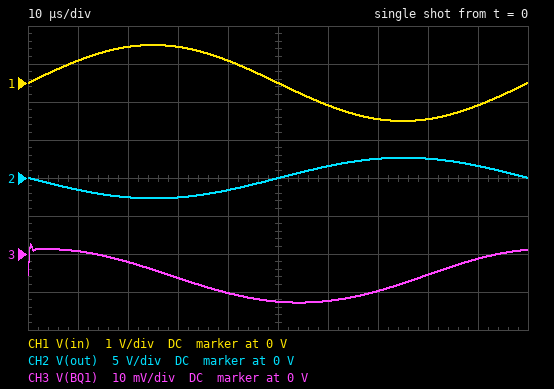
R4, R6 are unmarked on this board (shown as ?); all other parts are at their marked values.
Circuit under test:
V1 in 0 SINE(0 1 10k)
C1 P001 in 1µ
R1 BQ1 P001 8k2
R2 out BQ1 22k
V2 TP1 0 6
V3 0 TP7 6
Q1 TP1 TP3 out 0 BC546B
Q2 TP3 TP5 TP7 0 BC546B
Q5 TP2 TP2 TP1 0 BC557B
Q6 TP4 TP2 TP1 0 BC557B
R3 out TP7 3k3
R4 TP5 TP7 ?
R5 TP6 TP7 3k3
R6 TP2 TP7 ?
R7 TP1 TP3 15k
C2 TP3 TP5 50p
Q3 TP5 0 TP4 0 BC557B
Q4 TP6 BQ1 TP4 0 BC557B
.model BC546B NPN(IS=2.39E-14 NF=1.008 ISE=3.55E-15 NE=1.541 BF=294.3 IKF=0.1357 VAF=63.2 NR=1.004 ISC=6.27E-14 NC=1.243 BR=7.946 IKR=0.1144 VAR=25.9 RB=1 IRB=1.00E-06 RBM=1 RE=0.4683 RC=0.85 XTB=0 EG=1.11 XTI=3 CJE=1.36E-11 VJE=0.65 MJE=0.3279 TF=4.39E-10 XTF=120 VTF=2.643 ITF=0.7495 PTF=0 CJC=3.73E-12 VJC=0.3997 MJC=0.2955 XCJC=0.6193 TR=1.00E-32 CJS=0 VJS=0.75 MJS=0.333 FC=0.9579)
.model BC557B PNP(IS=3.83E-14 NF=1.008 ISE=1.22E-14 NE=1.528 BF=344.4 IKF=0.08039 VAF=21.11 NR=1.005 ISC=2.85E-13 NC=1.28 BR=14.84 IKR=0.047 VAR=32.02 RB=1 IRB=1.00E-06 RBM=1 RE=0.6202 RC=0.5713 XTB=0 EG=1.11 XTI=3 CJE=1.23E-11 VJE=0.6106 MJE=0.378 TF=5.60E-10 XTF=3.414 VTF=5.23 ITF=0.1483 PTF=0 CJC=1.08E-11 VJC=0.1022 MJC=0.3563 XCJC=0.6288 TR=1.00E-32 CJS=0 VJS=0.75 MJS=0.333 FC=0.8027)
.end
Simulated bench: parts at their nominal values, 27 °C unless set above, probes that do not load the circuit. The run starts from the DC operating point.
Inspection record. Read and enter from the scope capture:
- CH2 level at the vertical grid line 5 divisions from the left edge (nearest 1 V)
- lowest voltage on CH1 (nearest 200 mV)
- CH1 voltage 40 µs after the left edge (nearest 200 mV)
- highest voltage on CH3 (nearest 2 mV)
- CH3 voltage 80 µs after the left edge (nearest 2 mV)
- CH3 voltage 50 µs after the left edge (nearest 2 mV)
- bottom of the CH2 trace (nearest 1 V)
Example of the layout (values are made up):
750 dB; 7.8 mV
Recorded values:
0 V; -1.0 V; 600 mV; 2 mV; -6 mV; -12 mV; -3 V
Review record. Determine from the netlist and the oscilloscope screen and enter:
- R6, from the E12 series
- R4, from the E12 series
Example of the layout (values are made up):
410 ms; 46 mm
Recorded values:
100 kΩ; 10 kΩ
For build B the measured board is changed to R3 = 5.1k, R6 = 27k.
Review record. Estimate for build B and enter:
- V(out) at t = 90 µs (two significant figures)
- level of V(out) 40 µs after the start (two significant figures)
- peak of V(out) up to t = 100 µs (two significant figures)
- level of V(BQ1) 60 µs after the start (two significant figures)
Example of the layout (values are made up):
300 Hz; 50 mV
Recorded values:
1.5 V; -1.7 V; 2.6 V; -58 mV
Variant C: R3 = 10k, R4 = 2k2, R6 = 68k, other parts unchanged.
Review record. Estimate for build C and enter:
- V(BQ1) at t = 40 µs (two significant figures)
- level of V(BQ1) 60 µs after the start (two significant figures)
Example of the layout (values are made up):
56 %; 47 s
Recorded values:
5.7 V; 4.9 V
